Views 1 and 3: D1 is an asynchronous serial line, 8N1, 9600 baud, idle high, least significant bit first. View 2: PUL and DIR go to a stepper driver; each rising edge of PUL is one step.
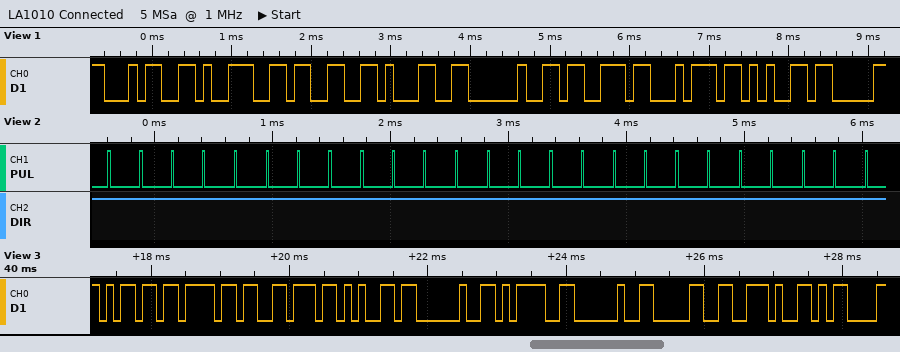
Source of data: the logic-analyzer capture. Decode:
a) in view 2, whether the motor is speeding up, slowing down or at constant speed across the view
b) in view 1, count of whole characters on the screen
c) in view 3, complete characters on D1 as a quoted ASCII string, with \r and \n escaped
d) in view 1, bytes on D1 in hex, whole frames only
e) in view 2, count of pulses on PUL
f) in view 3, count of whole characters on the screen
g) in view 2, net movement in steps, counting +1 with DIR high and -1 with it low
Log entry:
constant speed
8
"move = 0.\r"
34 39 33 31 20 73 74 65
25
10
+25
